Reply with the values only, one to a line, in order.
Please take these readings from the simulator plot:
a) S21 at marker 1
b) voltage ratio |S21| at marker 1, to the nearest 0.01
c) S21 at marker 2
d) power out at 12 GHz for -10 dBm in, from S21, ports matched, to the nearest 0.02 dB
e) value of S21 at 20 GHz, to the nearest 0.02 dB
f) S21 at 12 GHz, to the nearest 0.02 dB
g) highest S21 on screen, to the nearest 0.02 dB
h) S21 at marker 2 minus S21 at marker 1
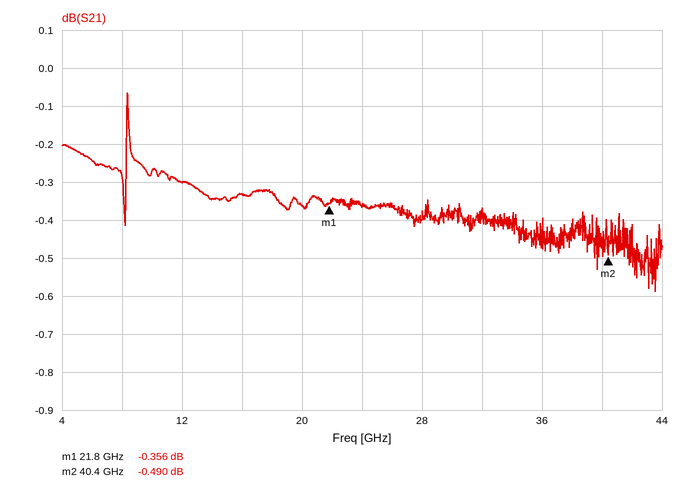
-0.356 dB
0.96
-0.490 dB
-10.30 dBm
-0.36 dB
-0.30 dB
-0.06 dB
-0.134 dB
